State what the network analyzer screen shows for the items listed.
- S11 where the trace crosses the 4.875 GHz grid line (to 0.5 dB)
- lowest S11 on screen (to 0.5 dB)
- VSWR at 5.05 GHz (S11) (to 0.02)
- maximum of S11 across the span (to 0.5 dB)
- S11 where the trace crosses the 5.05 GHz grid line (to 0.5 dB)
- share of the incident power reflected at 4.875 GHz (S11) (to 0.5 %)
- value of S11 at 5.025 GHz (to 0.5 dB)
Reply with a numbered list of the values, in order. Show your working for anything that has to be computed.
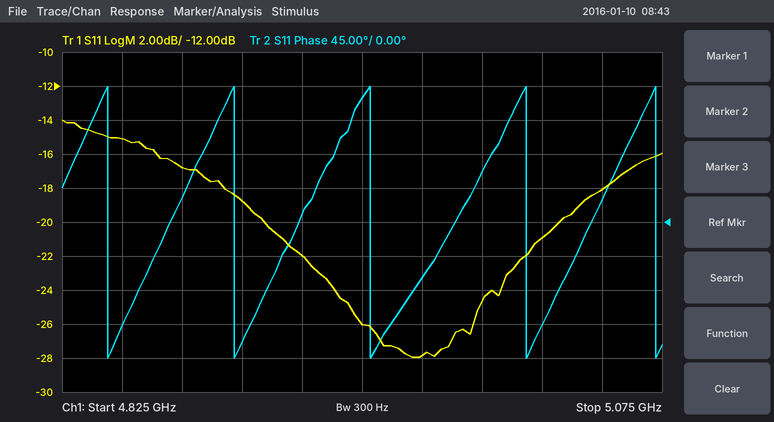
1. -17.0 dB
2. -28.0 dB
3. |Γ| = 10^(-18/20) = 0.1259; VSWR = (1 + 0.1259)/(1 − 0.1259) ≈ 1.29, so 1.28 to the nearest 0.02
4. -14.0 dB
5. -18.0 dB
6. 10^(-17/10) ≈ 2.0 %
7. -21.0 dB
